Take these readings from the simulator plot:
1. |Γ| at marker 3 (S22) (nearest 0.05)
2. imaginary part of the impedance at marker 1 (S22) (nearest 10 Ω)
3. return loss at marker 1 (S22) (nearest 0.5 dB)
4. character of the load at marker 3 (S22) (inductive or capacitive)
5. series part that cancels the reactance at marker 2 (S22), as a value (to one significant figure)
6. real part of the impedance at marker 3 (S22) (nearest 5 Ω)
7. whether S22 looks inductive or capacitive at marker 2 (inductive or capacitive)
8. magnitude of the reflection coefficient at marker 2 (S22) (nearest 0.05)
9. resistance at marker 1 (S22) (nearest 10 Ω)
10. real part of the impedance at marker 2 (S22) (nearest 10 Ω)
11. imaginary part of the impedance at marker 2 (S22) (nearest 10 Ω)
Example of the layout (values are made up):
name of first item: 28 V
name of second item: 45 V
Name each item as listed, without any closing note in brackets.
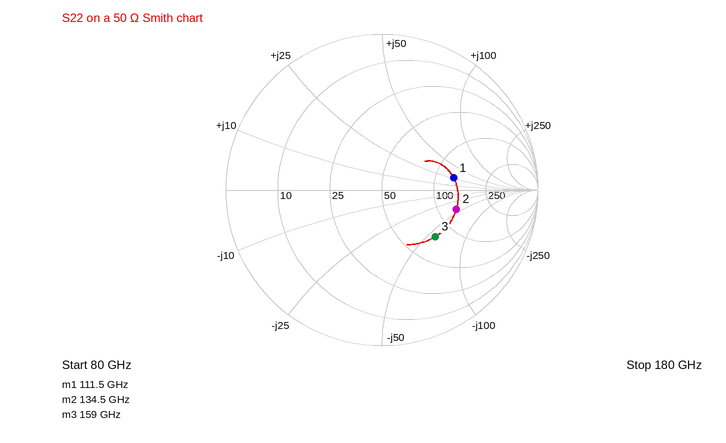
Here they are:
|Γ| at marker 3 (S22): 0.45
imaginary part of the impedance at marker 1 (S22): +30 Ω
return loss at marker 1 (S22): 6.5 dB
character of the load at marker 3 (S22): capacitive
series part that cancels the reactance at marker 2 (S22), as a value: 50 pH
real part of the impedance at marker 3 (S22): 75 Ω
whether S22 looks inductive or capacitive at marker 2: capacitive
magnitude of the reflection coefficient at marker 2 (S22): 0.50
resistance at marker 1 (S22): 130 Ω
real part of the impedance at marker 2 (S22): 130 Ω
imaginary part of the impedance at marker 2 (S22): -40 Ω
